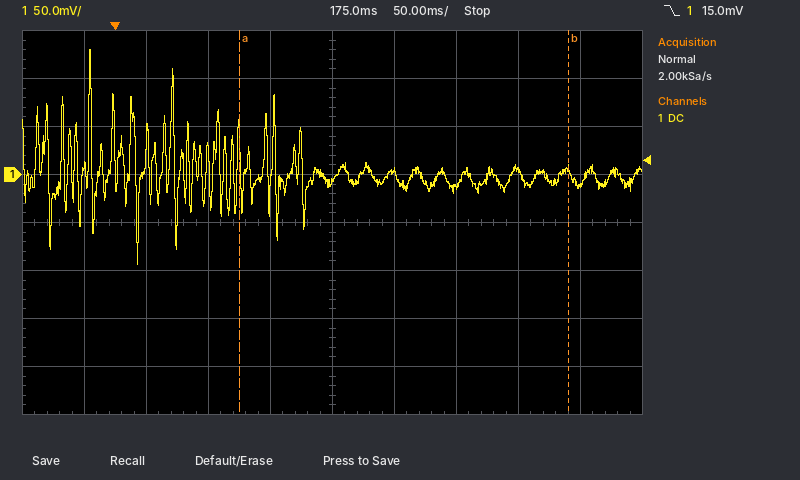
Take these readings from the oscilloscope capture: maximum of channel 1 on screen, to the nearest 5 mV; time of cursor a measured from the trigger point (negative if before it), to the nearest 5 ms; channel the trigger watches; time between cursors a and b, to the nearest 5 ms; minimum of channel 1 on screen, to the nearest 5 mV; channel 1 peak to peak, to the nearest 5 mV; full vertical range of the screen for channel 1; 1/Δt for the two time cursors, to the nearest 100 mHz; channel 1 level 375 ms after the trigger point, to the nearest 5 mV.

130 mV
+100 ms
channel 1
265 ms
-95 mV
225 mV
400 mV
3.8 Hz
-10 mV
